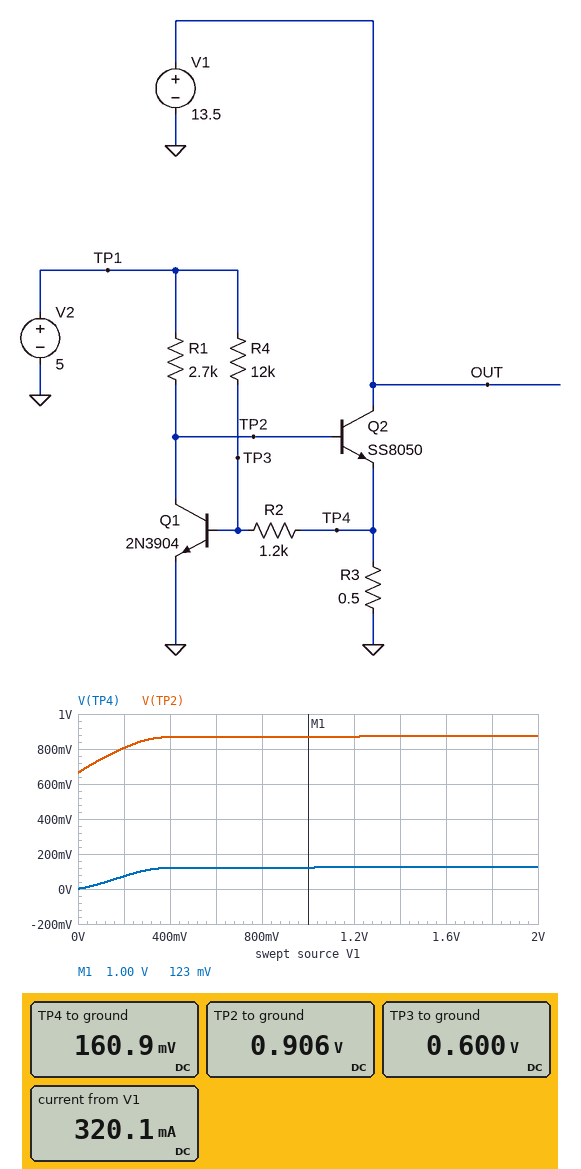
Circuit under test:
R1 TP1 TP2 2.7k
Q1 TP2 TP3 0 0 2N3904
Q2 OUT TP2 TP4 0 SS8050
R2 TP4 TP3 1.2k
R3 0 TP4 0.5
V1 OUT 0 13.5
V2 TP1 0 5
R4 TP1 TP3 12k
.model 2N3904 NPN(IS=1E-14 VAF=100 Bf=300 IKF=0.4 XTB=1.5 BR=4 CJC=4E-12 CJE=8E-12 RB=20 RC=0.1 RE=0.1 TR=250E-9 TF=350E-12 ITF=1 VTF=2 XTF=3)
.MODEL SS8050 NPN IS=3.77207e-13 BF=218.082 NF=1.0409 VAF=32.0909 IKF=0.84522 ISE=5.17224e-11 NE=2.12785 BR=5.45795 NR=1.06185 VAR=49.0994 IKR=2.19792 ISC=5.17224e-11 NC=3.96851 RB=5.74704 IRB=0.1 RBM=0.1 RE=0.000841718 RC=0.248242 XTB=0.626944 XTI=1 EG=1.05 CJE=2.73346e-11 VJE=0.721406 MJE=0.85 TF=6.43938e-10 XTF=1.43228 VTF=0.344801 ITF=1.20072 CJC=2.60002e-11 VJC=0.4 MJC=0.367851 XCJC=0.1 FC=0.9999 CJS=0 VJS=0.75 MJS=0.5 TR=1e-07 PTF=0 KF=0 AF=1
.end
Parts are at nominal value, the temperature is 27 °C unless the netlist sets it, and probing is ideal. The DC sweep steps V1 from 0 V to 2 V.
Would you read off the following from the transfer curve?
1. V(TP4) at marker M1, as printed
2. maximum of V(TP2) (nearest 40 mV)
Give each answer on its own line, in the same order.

123 mV
880 mV
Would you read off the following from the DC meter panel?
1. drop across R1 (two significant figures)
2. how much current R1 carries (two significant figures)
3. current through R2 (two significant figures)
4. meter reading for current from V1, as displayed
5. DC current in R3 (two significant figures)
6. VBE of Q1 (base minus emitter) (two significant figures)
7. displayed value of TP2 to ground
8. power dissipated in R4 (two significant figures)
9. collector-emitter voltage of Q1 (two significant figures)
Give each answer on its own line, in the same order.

4.1 V
1.5 mA
370 µA
320.1 mA
320 mA
600 mV
0.906 V
1.6 mW
910 mV
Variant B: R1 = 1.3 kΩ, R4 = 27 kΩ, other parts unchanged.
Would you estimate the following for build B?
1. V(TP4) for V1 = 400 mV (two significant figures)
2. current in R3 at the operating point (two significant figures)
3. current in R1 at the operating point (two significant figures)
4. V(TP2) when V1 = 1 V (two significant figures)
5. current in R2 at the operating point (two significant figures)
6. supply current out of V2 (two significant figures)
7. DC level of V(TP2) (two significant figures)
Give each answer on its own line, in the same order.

180 mV
590 mA
3.0 mA
990 mV
170 µA
3.2 mA
1.1 V
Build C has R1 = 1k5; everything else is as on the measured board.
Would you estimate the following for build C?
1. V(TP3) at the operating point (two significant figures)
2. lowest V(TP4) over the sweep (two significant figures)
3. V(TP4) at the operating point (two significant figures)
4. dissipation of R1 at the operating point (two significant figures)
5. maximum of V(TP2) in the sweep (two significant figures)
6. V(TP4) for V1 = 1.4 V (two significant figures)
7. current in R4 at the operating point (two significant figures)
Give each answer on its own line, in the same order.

650 mV
3.2 mV
210 mV
11 mW
950 mV
180 mV
360 µA
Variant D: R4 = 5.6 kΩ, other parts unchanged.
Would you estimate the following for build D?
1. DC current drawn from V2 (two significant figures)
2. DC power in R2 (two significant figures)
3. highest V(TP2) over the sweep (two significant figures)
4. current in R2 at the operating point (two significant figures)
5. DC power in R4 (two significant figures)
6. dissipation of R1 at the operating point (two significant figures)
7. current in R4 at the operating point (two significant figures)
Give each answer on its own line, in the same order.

2.6 mA
390 µW
34 mV
570 µA
3.3 mW
9.1 mW
770 µA
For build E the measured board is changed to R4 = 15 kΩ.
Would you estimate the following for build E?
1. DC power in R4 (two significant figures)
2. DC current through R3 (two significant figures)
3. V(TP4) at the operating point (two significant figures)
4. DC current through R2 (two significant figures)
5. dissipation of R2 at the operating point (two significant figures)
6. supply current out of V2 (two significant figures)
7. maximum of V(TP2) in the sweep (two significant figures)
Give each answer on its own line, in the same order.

1.3 mW
340 mA
170 mV
300 µA
110 µW
1.8 mA
880 mV
